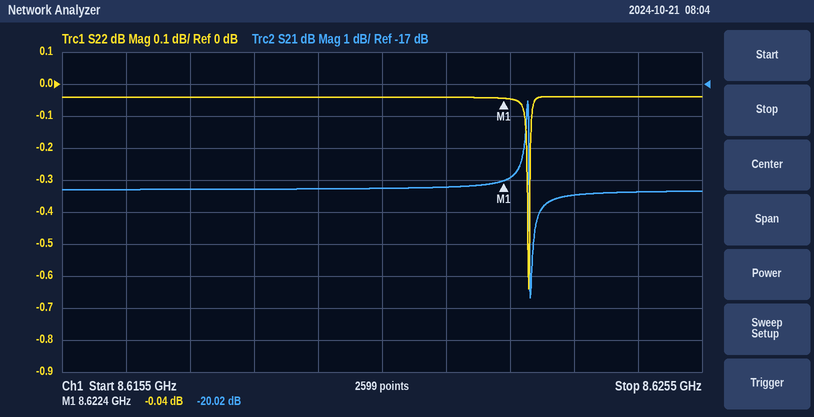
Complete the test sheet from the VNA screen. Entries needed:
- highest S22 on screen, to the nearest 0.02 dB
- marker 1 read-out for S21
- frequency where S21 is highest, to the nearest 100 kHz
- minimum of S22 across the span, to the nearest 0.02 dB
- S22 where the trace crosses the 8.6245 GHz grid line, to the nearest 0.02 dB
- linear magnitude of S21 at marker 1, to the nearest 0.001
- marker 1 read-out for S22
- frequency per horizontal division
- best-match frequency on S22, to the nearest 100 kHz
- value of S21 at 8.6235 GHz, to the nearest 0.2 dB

-0.04 dB
-20.02 dB
8.6228 GHz
-0.64 dB
-0.04 dB
0.100
-0.04 dB
1 MHz
8.6228 GHz
-20.4 dB
